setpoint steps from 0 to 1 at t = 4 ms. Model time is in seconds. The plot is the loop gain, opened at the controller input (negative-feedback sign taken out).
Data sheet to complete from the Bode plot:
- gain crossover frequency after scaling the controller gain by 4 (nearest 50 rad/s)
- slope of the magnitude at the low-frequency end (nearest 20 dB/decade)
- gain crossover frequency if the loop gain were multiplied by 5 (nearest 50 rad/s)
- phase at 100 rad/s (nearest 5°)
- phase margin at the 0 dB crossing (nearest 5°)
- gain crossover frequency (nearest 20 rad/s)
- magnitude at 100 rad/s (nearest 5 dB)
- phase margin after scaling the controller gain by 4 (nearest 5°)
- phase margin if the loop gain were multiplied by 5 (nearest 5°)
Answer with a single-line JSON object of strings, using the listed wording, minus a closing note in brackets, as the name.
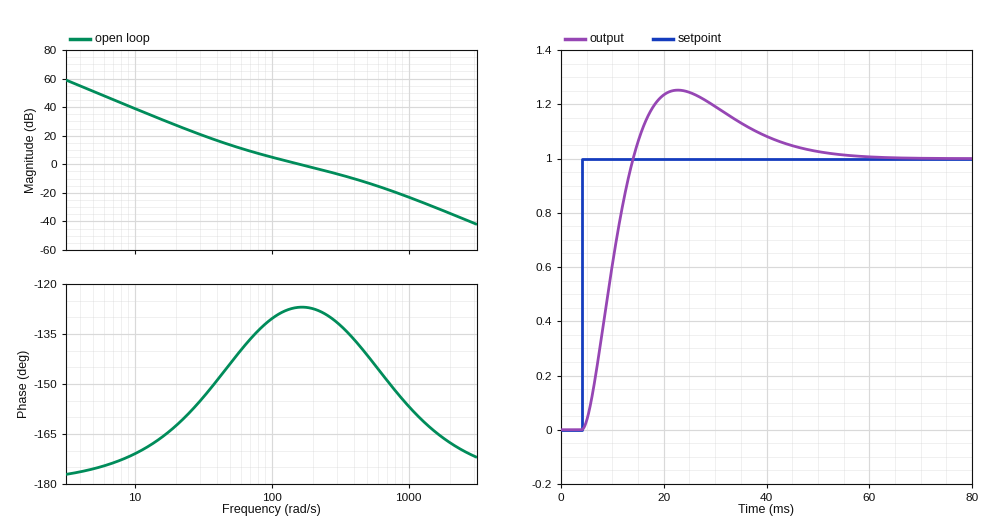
{"gain crossover frequency after scaling the controller gain by 4": "450 rad/s", "slope of the magnitude at the low-frequency end": "-40 dB/decade", "gain crossover frequency if the loop gain were multiplied by 5": "550 rad/s", "phase at 100 rad/s": "-130°", "phase margin at the 0 dB crossing": "55°", "gain crossover frequency": "160 rad/s", "magnitude at 100 rad/s": "5 dB", "phase margin after scaling the controller gain by 4": "40°", "phase margin if the loop gain were multiplied by 5": "35°"}
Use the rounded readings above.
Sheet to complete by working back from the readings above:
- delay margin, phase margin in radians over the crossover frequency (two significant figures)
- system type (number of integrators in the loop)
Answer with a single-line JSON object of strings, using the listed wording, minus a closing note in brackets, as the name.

{"delay margin, phase margin in radians over the crossover frequency": "0.0060 s", "system type": "2"}
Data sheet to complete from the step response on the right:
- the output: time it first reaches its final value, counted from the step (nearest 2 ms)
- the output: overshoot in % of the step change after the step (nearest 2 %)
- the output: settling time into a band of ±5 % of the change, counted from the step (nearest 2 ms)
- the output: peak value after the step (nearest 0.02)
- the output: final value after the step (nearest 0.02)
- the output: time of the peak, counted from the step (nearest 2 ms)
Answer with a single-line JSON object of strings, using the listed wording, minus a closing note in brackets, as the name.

{"the output: time it first reaches its final value, counted from the step": "10 ms", "the output: overshoot in % of the step change after the step": "26 %", "the output: settling time into a band of ±5 % of the change, counted from the step": "40 ms", "the output: peak value after the step": "1.26", "the output: final value after the step": "1.00", "the output: time of the peak, counted from the step": "18 ms"}
